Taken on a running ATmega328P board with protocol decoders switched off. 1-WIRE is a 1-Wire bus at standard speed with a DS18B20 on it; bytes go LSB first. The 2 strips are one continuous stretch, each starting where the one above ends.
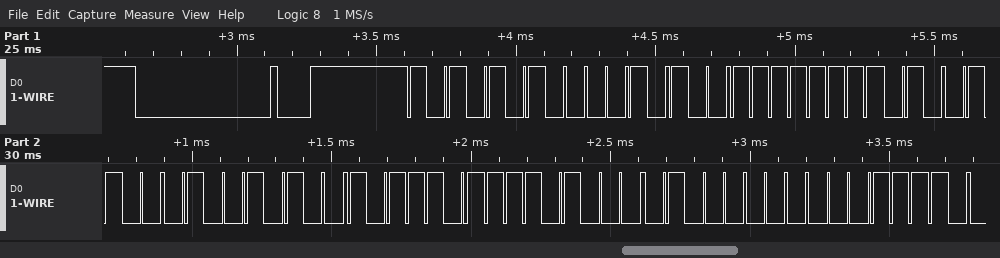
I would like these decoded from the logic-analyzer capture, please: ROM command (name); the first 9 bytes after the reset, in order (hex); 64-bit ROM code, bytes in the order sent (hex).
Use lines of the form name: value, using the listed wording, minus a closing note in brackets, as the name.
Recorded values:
ROM command: Match ROM
the first 9 bytes after the reset, in order: 55 28 FF 32 52 BA 17 02 78
64-bit ROM code, bytes in the order sent: 28 FF 32 52 BA 17 02 78
